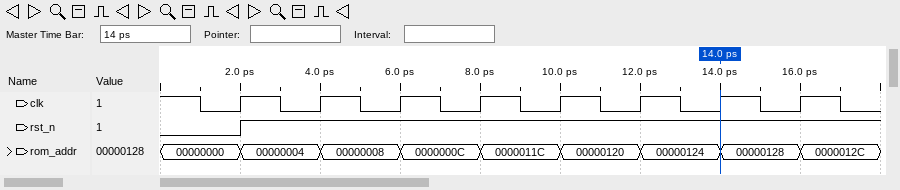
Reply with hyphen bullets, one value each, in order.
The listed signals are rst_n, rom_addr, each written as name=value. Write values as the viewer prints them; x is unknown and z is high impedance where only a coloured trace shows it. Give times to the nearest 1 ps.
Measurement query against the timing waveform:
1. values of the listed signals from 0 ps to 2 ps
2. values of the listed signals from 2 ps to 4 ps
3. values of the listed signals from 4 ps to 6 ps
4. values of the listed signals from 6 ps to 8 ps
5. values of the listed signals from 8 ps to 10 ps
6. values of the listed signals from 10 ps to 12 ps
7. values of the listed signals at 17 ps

- rst_n=0, rom_addr=00000000
- rst_n=1, rom_addr=00000004
- rst_n=1, rom_addr=00000008
- rst_n=1, rom_addr=0000000C
- rst_n=1, rom_addr=0000011C
- rst_n=1, rom_addr=00000120
- rst_n=1, rom_addr=0000012C
